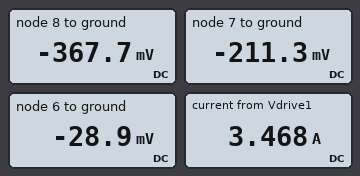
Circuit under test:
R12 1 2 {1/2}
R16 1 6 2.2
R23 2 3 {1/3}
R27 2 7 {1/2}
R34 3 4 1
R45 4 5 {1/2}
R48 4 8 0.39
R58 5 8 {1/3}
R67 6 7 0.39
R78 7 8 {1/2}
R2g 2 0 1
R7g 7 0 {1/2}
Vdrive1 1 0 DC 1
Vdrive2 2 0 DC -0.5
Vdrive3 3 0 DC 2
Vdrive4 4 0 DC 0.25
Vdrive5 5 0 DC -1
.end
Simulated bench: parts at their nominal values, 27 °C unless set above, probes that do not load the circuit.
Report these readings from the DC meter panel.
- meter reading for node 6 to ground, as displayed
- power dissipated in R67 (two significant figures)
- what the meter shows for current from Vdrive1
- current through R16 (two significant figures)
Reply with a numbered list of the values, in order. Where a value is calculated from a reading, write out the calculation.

1. -28.9 mV
2. (-28.9 mV - (-211.3 mV))^2 / 390 mΩ = 85 mW
3. 3.468 A
4. (1 V - (-28.9 mV)) / 2.2 Ω = 470 mA
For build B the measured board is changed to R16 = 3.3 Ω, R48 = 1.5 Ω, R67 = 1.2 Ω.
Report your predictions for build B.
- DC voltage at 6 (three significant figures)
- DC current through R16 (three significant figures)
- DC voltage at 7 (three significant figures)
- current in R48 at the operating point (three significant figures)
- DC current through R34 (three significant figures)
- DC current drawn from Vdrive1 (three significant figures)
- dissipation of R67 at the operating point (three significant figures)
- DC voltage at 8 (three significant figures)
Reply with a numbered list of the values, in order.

1. 30.3 mV
2. 294 mA
3. -322 mV
4. 576 mA
5. 1.75 A
6. 3.29 A
7. 104 mW
8. -614 mV
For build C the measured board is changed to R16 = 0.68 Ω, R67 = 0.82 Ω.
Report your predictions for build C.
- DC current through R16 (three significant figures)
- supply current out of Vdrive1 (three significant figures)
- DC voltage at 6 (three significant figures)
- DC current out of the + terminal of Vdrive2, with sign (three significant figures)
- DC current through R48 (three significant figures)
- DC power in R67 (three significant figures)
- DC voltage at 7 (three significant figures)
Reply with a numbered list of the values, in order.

1. 771 mA
2. 3.77 A
3. 476 mV
4. -11.7 A
5. 1.55 A
6. 487 mW
7. -156 mV
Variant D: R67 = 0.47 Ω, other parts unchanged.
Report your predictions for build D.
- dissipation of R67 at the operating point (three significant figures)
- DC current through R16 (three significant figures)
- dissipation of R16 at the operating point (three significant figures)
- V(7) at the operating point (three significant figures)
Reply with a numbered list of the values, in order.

1. 97.1 mW
2. 455 mA
3. 455 mW
4. -214 mV
